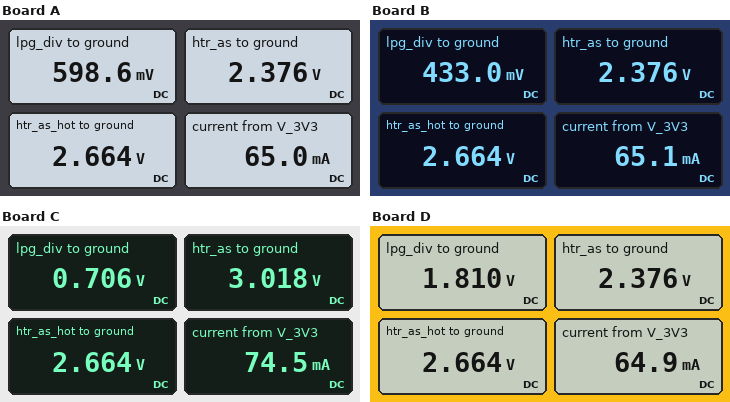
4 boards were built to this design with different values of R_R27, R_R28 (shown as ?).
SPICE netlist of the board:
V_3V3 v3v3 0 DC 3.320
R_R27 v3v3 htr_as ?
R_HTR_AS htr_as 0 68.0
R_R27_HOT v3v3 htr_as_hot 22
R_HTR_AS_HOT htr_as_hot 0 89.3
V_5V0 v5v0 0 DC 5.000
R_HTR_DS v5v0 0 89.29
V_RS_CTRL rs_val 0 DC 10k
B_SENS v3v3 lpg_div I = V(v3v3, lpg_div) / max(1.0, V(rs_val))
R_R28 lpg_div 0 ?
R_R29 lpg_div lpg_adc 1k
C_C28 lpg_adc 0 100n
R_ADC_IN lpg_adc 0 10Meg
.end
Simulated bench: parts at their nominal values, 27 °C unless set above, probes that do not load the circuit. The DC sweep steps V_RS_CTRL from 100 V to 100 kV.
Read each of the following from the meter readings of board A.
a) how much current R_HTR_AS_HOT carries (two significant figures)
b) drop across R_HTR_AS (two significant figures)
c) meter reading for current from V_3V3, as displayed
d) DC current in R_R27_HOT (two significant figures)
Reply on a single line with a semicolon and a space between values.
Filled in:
30 mA; 2.4 V; 65.0 mA; 30 mA
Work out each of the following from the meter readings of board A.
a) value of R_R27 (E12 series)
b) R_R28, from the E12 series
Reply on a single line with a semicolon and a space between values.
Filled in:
27 Ω; 2.2 kΩ
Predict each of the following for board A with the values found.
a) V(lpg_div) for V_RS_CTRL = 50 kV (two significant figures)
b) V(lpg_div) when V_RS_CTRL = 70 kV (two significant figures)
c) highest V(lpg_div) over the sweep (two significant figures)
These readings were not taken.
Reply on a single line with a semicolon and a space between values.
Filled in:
140 mV; 100 mV; 3.2 V
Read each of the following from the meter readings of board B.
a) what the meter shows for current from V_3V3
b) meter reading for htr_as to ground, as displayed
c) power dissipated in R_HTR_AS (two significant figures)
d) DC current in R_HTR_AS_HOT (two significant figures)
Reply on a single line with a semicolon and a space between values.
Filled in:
65.1 mA; 2.376 V; 83 mW; 30 mA
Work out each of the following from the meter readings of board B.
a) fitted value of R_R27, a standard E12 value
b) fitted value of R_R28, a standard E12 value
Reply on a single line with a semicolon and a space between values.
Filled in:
27 Ω; 1.5 kΩ
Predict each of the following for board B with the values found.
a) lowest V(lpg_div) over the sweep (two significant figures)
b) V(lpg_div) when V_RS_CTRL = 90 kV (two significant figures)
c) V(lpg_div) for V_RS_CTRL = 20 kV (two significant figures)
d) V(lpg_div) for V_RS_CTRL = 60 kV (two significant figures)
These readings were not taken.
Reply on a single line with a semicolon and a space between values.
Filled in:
49 mV; 54 mV; 230 mV; 81 mV
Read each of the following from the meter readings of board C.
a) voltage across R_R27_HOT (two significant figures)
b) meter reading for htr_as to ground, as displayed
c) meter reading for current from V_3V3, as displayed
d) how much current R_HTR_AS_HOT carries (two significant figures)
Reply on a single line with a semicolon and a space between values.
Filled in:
660 mV; 3.018 V; 74.5 mA; 30 mA
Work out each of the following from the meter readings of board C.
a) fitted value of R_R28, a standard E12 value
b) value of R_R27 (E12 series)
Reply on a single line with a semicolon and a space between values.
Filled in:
2.7 kΩ; 6.8 Ω
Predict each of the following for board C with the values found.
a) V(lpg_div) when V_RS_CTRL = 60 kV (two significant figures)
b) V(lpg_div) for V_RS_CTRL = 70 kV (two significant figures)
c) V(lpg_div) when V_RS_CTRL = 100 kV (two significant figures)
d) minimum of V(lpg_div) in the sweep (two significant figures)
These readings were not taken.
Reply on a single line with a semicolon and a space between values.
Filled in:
140 mV; 120 mV; 87 mV; 87 mV
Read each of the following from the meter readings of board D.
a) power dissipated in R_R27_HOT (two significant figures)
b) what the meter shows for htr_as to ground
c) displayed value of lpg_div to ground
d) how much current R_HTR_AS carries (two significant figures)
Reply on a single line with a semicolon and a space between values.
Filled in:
20 mW; 2.376 V; 1.810 V; 35 mA
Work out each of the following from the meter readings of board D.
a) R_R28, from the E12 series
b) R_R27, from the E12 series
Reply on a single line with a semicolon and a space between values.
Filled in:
12 kΩ; 27 Ω
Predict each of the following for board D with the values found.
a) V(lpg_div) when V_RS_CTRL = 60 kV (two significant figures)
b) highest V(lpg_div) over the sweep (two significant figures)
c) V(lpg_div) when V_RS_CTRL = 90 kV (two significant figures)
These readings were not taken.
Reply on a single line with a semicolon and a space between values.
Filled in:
550 mV; 3.3 V; 390 mV
